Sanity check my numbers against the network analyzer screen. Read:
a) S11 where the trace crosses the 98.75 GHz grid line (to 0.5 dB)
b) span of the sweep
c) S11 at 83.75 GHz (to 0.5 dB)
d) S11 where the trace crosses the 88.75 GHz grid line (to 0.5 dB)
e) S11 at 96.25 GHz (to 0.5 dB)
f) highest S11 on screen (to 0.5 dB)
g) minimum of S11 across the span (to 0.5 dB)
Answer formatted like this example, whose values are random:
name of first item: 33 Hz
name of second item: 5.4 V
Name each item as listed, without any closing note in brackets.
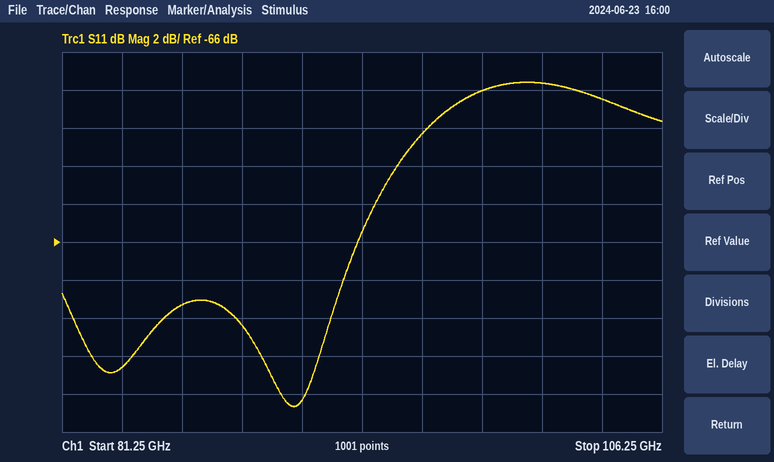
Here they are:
S11 where the trace crosses the 98.75 GHz grid line: -58.0 dB
span of the sweep: 25 GHz
S11 at 83.75 GHz: -72.5 dB
S11 where the trace crosses the 88.75 GHz grid line: -70.5 dB
S11 at 96.25 GHz: -60.5 dB
highest S11 on screen: -57.5 dB
minimum of S11 across the span: -74.5 dB
